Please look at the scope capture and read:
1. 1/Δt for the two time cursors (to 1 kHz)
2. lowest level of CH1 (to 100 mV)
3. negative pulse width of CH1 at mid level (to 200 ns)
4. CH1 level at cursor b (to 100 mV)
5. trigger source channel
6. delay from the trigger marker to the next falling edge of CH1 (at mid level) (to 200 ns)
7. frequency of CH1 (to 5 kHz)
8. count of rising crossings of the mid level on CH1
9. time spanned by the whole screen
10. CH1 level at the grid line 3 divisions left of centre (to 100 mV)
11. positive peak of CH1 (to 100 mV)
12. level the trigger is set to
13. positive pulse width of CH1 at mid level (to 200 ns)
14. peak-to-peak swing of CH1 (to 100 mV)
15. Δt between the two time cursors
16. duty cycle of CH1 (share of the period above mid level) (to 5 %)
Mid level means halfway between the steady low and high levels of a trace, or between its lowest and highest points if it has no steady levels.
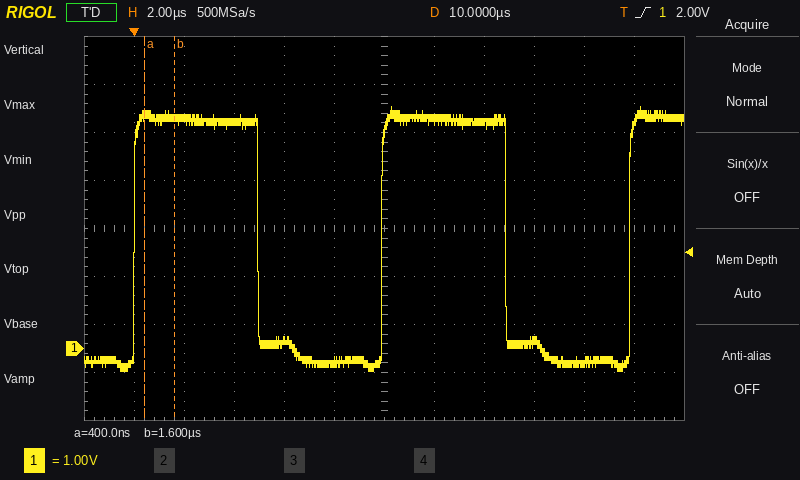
833 kHz
-500 mV
5.0 µs
4.8 V
CH1
5.0 µs
100 kHz
3
24 µs
4.7 V
5.0 V
2.00 V
5.0 µs
5.5 V
1.2 µs
50 %
